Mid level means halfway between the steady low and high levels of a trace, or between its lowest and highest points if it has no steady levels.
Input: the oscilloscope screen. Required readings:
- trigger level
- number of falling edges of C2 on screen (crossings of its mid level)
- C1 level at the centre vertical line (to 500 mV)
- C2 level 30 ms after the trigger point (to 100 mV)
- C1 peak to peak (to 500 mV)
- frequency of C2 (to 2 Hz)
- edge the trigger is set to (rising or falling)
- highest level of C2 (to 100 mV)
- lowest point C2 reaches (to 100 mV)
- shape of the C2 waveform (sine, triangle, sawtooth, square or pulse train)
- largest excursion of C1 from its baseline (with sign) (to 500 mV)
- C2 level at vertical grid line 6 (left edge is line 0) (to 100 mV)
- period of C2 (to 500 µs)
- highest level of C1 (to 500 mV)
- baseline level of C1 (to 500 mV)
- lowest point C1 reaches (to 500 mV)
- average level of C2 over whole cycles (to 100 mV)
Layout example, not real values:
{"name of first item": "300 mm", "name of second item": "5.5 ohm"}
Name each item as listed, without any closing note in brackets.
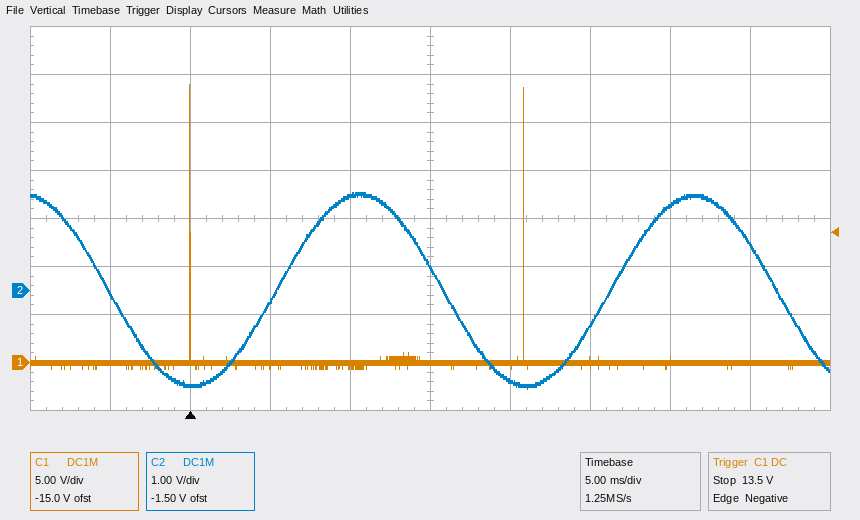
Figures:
{"trigger level": "13.5 V", "number of falling edges of C2 on screen": "3", "C1 level at the centre vertical line": "0.0 V", "C2 level 30 ms after the trigger point": "1.8 V", "C1 peak to peak": "29.5 V", "frequency of C2": "48 Hz", "edge the trigger is set to": "falling", "highest level of C2": "2.0 V", "lowest point C2 reaches": "-2.0 V", "shape of the C2 waveform": "sine", "largest excursion of C1 from its baseline (with sign)": "+29.0 V", "C2 level at vertical grid line 6 (left edge is line 0)": "-1.9 V", "period of C2": "21.0 ms", "highest level of C1": "29.0 V", "baseline level of C1": "0.0 V", "lowest point C1 reaches": "-500 mV", "average level of C2 over whole cycles": "0.0 V"}
